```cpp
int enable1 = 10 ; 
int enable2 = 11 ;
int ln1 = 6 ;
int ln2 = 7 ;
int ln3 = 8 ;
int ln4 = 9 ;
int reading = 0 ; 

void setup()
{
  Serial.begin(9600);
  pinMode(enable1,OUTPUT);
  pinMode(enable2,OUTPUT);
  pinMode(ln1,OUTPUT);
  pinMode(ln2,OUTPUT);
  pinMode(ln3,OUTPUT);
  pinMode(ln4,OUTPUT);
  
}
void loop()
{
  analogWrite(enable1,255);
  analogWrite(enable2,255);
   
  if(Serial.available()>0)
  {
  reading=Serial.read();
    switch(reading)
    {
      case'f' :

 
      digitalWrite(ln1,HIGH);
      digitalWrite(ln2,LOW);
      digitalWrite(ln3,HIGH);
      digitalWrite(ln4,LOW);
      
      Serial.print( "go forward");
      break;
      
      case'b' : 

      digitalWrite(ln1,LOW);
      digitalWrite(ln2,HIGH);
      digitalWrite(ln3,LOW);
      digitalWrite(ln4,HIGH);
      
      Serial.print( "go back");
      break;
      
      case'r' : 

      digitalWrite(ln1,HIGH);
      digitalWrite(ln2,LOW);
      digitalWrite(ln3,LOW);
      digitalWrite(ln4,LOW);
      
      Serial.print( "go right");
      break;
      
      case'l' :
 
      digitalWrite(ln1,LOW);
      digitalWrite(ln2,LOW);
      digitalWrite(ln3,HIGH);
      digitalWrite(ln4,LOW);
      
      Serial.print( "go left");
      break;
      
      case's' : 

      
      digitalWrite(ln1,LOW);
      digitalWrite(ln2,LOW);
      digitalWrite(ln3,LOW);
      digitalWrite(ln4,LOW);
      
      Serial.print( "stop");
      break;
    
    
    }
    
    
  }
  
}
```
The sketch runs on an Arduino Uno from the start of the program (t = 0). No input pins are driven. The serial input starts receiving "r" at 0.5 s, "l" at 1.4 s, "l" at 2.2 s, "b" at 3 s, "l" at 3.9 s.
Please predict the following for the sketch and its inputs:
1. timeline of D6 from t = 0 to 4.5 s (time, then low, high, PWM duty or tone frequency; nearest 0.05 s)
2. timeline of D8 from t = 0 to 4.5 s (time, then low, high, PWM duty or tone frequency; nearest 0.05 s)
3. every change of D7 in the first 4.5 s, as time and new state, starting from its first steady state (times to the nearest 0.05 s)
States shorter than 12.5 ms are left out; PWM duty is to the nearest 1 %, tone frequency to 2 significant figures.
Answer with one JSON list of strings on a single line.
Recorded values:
["0 s low; 0.5 s high; 1.4 s low", "0 s low; 1.4 s high; 3 s low; 3.9 s high", "0 s low; 3 s high; 3.9 s low"]
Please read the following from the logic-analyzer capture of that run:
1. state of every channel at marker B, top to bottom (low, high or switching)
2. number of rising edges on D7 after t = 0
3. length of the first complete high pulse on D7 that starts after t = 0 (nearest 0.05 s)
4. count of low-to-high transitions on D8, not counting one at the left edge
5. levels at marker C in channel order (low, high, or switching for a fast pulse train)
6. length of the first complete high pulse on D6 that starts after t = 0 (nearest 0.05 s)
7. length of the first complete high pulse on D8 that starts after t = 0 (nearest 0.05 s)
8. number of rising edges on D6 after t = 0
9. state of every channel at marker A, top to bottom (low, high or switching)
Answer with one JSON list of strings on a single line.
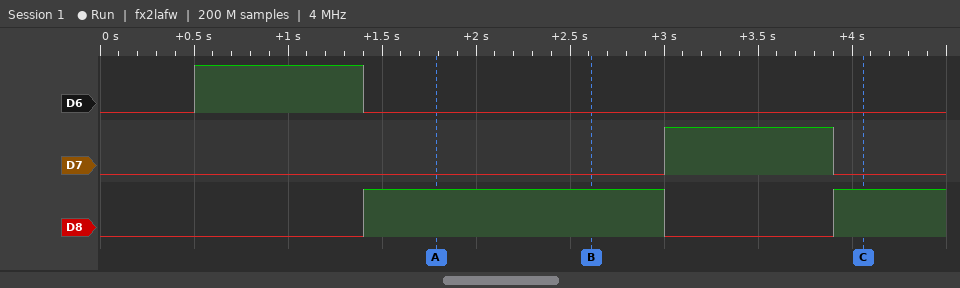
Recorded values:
["D6 low, D7 low, D8 high", "1", "0.90 s", "2", "D6 low, D7 low, D8 high", "0.90 s", "1.60 s", "1", "D6 low, D7 low, D8 high"]
